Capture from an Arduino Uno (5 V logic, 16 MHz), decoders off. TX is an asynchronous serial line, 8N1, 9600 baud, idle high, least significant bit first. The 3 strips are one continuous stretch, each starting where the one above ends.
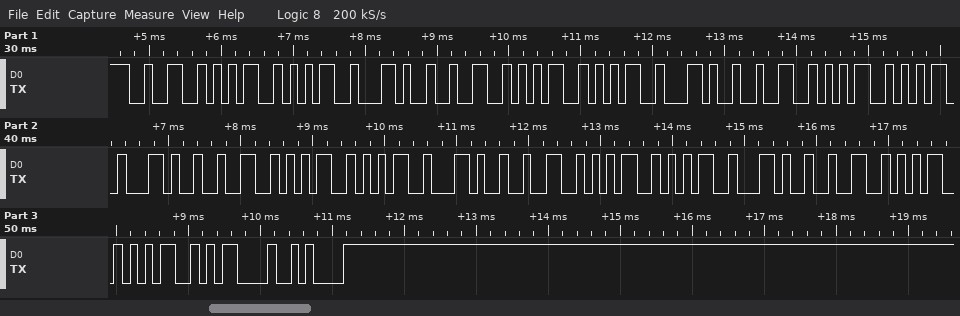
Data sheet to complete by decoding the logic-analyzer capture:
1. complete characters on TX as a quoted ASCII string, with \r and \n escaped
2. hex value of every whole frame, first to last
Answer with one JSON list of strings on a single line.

["\"255,255,255,255,255,255\\r\\n\"", "32 35 35 2C 32 35 35 2C 32 35 35 2C 32 35 35 2C 32 35 35 2C 32 35 35 0D 0A"]
